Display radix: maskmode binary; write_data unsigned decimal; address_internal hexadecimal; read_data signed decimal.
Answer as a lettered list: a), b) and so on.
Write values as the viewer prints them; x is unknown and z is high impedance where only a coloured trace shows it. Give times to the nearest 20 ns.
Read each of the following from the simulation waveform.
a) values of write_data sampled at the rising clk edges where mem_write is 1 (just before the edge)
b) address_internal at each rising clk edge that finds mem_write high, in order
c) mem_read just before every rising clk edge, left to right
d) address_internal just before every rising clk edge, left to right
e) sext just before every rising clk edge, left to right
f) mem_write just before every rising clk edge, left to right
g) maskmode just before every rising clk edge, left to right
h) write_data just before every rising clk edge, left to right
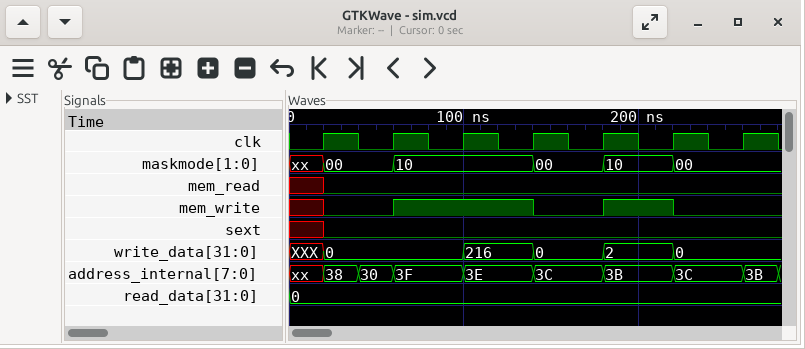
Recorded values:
a) 0, 216, 2
b) 3F, 3E, 3B
c) x 0 0 0 0 0 0
d) xx, 30, 3F, 3E, 3C, 3B, 3C
e) x 0 0 0 0 0 0
f) x 0 1 1 0 1 0
g) xx, 00, 10, 10, 00, 10, 00
h) XXX, 0, 0, 216, 0, 2, 0
